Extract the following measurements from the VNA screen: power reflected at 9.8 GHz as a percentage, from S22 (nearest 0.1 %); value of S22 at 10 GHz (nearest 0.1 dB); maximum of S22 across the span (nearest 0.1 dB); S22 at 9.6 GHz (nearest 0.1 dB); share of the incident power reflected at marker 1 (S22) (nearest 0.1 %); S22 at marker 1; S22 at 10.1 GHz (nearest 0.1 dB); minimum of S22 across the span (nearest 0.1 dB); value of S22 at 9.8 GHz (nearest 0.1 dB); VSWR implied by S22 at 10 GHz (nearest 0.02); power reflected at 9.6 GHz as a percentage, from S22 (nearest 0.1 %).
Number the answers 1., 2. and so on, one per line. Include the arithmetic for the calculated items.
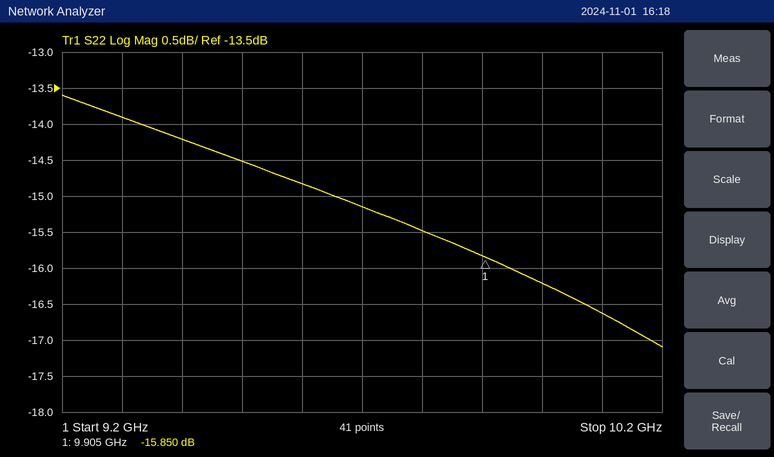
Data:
1. 10^(-15.5/10) ≈ 2.8 %
2. -16.2 dB
3. -13.6 dB
4. -14.8 dB
5. 10^(-15.85/10) ≈ 2.6 %
6. -15.850 dB
7. -16.6 dB
8. -17.1 dB
9. -15.5 dB
10. |Γ| = 10^(-16.2/20) = 0.1549; VSWR = (1 + 0.1549)/(1 − 0.1549) ≈ 1.37, so 1.36 to the nearest 0.02
11. 10^(-14.8/10) ≈ 3.3 %
